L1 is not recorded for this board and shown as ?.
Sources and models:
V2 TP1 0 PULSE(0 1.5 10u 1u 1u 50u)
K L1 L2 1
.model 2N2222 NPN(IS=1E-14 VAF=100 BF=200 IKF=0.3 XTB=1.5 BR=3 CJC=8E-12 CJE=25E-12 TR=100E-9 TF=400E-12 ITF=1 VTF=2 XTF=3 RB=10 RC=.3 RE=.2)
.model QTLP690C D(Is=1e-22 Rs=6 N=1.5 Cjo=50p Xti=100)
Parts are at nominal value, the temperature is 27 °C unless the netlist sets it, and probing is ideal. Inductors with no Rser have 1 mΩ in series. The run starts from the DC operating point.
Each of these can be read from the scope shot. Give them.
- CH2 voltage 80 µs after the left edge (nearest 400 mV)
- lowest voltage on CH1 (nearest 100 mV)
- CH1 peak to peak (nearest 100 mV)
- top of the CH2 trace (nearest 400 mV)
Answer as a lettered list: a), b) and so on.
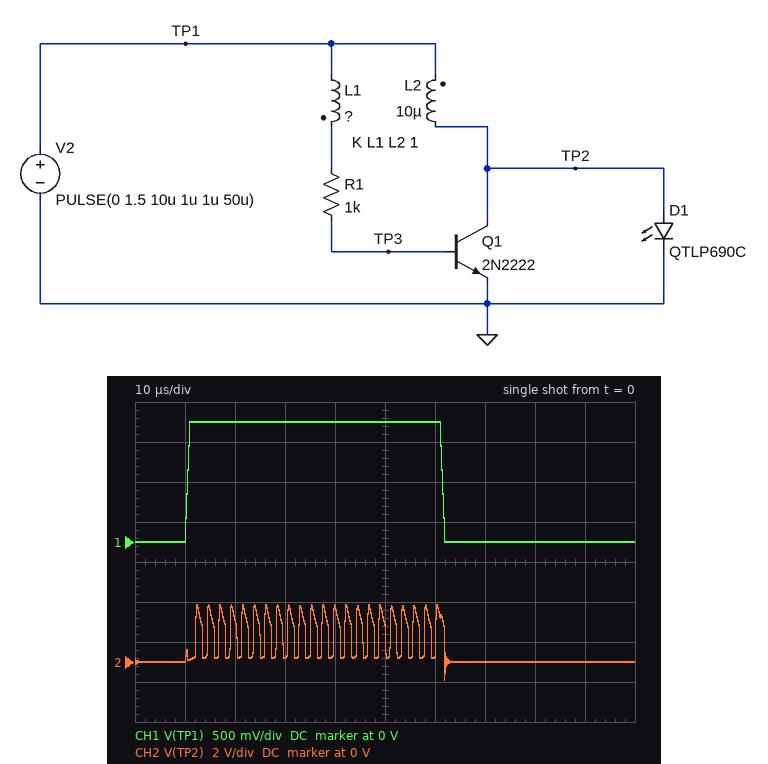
a) 0 V
b) 0 V
c) 1.5 V
d) 2.8 V
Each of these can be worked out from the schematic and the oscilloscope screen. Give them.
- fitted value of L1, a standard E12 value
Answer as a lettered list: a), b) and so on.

a) 3.3 µH
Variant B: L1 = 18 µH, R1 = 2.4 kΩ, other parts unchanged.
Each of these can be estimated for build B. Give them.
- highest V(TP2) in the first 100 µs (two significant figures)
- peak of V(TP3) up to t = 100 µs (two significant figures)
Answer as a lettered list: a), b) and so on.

a) 2.8 V
b) 840 mV
